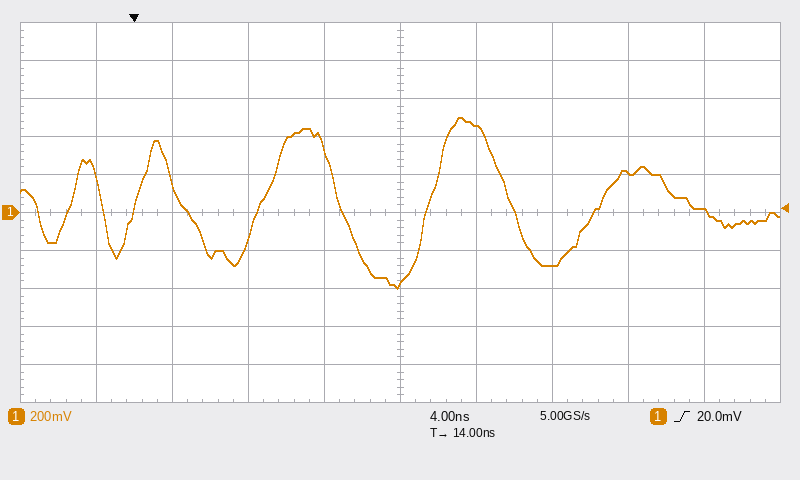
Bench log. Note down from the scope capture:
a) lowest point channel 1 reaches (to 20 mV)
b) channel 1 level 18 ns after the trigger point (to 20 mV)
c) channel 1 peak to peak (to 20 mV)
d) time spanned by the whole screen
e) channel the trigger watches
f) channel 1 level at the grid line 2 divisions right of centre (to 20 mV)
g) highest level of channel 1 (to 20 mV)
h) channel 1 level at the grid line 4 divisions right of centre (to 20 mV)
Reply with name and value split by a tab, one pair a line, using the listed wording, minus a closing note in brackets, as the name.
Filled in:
lowest point channel 1 reaches	-400 mV
channel 1 level 18 ns after the trigger point	460 mV
channel 1 peak to peak	900 mV
time spanned by the whole screen	40 ns
channel the trigger watches	channel 1
channel 1 level at the grid line 2 divisions right of centre	-280 mV
highest level of channel 1	500 mV
channel 1 level at the grid line 4 divisions right of centre	0 mV
